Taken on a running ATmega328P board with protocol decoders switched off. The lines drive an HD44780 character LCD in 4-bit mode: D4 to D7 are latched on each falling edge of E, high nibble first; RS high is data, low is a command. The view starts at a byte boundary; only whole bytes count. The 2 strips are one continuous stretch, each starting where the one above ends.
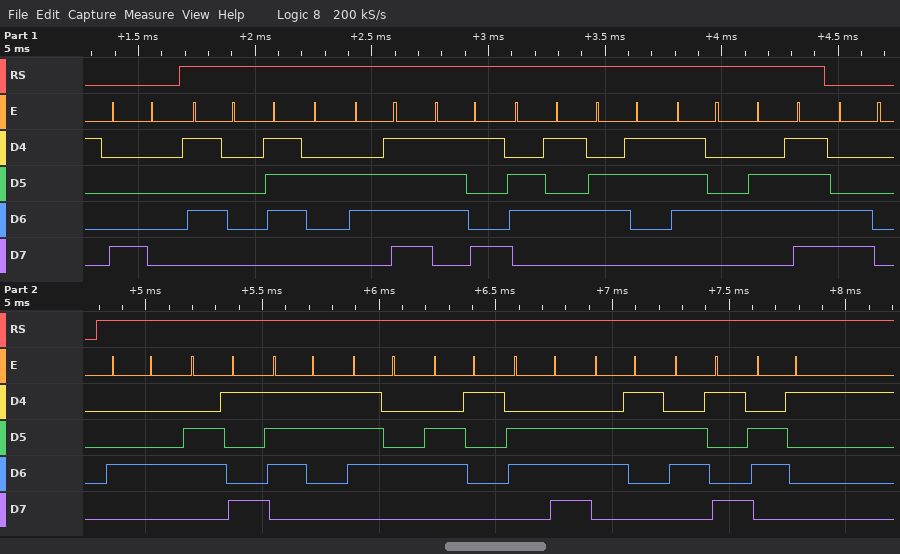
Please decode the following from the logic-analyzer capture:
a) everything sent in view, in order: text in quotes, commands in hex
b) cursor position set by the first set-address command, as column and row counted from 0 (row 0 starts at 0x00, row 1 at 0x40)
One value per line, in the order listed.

0x80 "Proyecto" 0xC0 "Distancia"
column 0, row 0
